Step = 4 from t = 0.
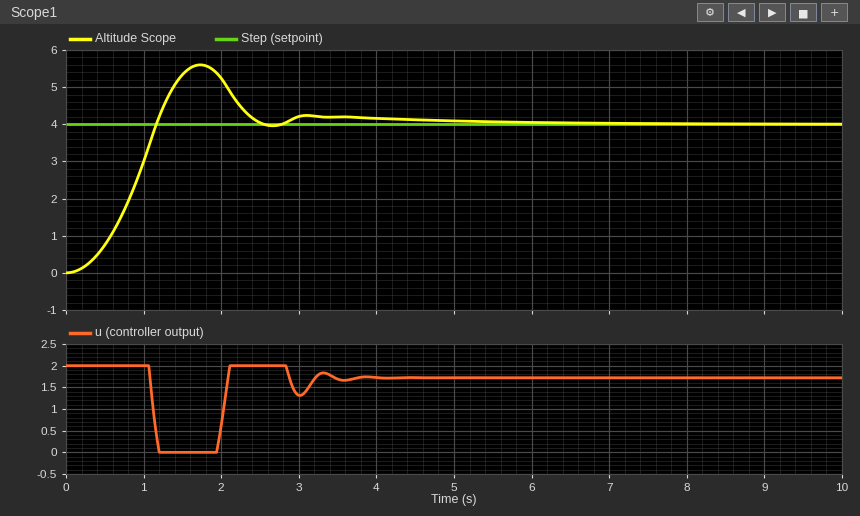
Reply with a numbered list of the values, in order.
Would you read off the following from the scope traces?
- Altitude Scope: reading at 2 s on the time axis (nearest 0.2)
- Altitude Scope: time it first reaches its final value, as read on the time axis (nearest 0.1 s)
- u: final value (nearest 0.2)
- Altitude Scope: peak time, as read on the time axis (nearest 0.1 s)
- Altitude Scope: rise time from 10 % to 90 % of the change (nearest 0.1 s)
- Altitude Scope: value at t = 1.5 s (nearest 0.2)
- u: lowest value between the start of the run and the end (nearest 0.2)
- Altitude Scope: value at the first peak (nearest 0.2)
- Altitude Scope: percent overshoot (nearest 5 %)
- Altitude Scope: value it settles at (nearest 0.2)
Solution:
1. 5.2
2. 1.2 s
3. 1.8
4. 1.7 s
5. 0.7 s
6. 5.4
7. 0.0
8. 5.6
9. 40 %
10. 4.0
